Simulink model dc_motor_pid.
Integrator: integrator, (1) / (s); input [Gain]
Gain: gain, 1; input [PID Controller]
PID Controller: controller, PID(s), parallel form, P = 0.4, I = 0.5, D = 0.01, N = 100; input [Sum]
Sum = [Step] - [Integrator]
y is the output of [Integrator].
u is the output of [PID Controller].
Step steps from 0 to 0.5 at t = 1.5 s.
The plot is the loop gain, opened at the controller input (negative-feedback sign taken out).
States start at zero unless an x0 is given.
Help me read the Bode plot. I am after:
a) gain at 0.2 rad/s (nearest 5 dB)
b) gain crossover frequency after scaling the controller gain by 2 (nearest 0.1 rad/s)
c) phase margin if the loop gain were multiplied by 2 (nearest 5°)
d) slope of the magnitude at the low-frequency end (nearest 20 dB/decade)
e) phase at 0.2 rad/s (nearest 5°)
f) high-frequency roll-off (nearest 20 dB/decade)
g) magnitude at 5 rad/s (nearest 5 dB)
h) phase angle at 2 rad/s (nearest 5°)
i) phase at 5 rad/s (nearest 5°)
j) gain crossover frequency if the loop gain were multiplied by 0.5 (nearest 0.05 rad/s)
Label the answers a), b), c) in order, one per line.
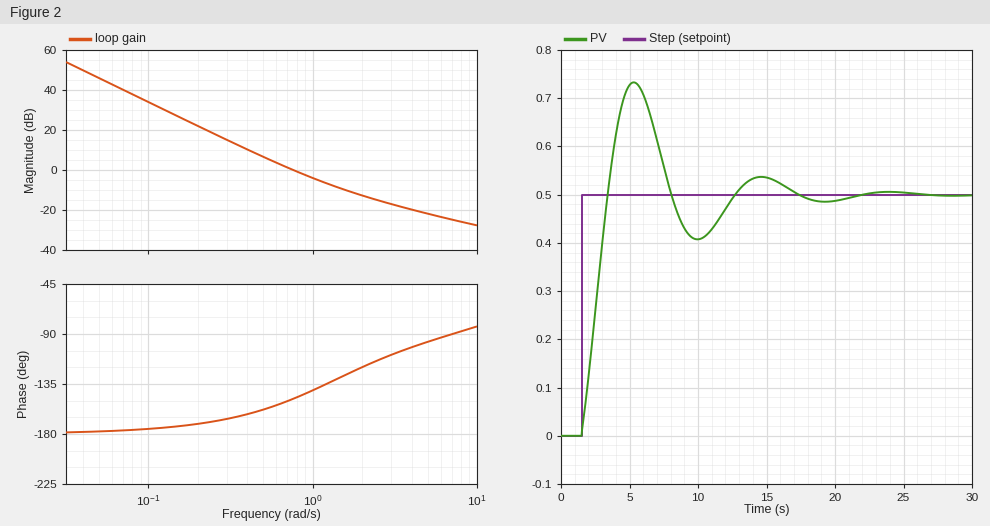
a) 20 dB
b) 1.2 rad/s
c) 45°
d) -40 dB/decade
e) -170°
f) -20 dB/decade
g) -20 dB
h) -120°
i) -95°
j) 0.50 rad/s
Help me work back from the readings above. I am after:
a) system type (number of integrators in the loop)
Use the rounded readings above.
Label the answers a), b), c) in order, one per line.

a) 2
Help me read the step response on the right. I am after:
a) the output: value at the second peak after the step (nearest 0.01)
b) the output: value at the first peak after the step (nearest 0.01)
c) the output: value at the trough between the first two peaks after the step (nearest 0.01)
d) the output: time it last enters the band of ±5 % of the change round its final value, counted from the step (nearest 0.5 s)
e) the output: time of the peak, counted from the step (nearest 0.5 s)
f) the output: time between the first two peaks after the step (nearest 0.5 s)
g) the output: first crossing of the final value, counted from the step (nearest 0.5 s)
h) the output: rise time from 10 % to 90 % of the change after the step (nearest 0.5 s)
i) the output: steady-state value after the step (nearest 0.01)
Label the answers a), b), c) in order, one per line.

a) 0.54
b) 0.73
c) 0.41
d) 14.5 s
e) 4.0 s
f) 9.5 s
g) 2.0 s
h) 1.5 s
i) 0.50
